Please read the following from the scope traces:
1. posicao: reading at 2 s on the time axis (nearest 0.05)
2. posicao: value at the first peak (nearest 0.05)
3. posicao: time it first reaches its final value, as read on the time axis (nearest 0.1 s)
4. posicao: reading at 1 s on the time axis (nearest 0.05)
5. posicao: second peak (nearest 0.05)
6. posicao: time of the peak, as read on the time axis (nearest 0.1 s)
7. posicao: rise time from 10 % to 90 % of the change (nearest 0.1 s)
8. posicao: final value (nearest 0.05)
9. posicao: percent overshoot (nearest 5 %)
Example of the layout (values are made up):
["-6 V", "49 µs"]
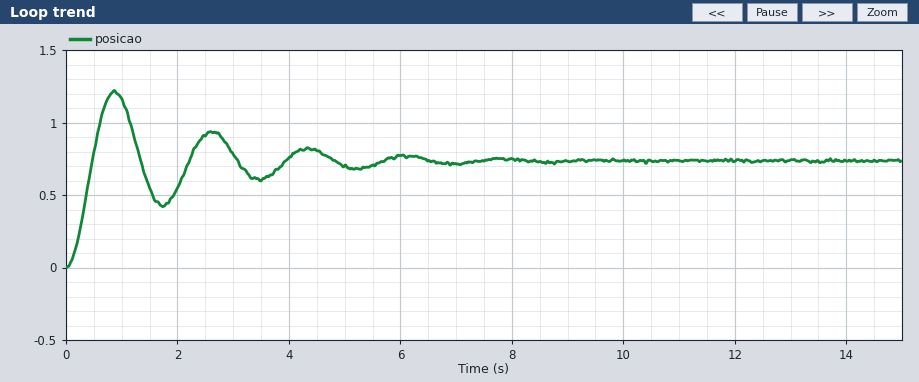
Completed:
["0.55", "1.20", "0.5 s", "1.15", "0.95", "0.9 s", "0.3 s", "0.75", "65 %"]
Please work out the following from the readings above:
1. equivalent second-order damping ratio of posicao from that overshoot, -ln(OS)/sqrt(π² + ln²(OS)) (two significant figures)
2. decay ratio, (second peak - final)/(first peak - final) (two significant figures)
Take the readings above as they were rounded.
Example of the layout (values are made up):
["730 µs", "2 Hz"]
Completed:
["0.14", "0.44"]
